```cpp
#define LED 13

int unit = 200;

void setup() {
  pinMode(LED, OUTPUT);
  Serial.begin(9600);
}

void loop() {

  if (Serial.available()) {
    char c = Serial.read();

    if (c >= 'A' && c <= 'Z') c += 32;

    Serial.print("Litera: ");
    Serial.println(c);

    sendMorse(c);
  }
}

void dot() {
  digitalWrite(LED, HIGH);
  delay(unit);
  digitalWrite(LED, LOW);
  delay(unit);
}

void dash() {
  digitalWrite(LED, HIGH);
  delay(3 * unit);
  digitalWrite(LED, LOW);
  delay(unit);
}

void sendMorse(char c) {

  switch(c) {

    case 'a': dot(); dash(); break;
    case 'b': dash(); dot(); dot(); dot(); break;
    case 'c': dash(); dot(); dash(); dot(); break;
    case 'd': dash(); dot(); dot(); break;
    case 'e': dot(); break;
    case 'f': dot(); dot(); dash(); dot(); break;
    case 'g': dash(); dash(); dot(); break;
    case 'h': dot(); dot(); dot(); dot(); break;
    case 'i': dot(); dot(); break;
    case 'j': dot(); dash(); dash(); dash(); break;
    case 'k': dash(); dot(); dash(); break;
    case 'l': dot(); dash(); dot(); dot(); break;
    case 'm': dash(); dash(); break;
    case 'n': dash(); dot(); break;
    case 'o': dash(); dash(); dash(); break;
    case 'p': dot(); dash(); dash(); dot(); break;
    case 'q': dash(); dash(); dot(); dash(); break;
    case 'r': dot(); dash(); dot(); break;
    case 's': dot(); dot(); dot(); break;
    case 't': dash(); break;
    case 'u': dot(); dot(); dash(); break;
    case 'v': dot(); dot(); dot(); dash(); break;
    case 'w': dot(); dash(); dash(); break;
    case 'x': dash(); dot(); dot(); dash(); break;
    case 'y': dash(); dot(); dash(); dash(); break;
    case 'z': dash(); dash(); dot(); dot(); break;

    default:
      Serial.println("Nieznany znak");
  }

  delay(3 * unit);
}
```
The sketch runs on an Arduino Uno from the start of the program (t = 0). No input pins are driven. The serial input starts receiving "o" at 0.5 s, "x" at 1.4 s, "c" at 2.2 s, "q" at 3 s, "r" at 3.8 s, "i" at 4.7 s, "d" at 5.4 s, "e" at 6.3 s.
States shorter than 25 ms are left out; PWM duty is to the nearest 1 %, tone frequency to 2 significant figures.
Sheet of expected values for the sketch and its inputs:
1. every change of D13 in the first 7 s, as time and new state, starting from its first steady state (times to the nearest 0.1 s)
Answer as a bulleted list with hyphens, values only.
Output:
- 0 s low; 0.5 s high; 1.1 s low; 1.3 s high; 1.9 s low; 2.1 s high; 2.7 s low; 3.5 s high; 4.1 s low; 4.3 s high; 4.5 s low; 4.7 s high; 4.9 s low; 5.1 s high; 5.7 s low; 6.5 s high
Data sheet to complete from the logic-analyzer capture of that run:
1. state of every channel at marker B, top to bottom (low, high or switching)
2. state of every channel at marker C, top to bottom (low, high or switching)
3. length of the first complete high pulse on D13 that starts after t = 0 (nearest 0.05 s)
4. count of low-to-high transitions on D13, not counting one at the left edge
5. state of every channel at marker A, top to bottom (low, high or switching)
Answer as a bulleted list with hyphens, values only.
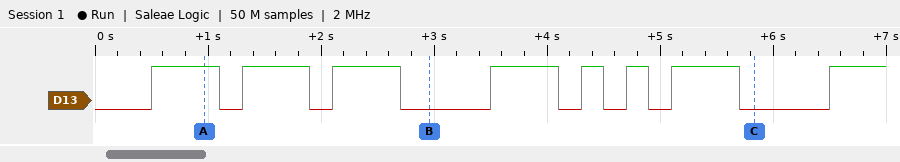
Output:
- D13 low
- D13 low
- 0.60 s
- 8
- D13 high
